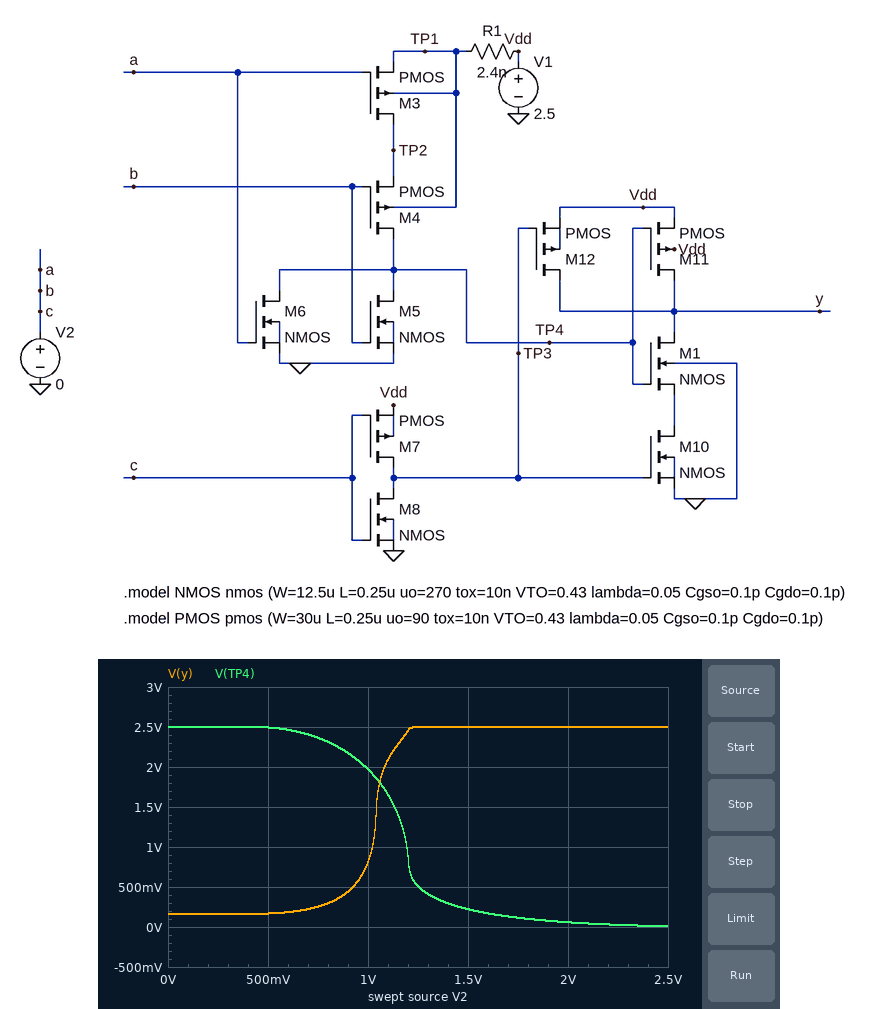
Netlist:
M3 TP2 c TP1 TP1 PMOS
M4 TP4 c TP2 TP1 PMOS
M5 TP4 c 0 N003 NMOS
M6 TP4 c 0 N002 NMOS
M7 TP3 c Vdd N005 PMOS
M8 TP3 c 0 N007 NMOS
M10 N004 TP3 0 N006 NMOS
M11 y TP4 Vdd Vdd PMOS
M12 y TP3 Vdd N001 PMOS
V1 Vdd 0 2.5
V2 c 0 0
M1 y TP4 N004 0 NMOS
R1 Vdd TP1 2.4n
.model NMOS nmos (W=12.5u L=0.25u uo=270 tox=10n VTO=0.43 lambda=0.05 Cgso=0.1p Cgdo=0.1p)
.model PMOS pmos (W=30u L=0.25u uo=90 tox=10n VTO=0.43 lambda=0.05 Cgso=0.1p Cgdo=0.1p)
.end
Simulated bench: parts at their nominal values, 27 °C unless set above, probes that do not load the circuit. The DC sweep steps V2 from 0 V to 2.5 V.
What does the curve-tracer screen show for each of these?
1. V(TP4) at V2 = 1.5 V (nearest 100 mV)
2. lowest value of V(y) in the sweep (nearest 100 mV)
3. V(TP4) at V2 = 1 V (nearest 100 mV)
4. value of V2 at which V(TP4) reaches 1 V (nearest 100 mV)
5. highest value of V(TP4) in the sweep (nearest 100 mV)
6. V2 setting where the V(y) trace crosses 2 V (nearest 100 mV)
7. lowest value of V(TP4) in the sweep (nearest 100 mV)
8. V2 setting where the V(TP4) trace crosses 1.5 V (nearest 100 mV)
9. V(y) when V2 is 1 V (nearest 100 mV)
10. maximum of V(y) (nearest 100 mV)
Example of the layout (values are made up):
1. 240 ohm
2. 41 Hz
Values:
1. 200 mV
2. 200 mV
3. 2.0 V
4. 1.2 V
5. 2.5 V
6. 1.1 V
7. 0 V
8. 1.1 V
9. 800 mV
10. 2.5 V
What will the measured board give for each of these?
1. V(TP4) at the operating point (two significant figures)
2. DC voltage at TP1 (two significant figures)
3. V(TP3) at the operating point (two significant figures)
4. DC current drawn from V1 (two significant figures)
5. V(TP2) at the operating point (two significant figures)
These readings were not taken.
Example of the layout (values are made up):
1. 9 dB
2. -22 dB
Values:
1. 2.5 V
2. 2.5 V
3. 2.5 V
4. 770 µA
5. 2.5 V
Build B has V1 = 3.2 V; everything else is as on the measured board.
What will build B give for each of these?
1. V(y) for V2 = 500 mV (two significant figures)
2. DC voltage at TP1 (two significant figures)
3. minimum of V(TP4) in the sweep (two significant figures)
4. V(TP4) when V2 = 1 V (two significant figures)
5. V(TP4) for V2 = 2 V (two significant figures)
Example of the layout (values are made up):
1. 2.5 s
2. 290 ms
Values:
1. 130 mV
2. 3.2 V
3. 67 mV
4. 2.8 V
5. 190 mV
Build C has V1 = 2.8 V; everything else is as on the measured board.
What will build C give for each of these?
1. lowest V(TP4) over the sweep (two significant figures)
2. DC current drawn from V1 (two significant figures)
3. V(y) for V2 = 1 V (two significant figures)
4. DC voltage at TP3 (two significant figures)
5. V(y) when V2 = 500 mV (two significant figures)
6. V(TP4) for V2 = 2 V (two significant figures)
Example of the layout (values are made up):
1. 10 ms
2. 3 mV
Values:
1. 28 mV
2. 780 µA
3. 510 mV
4. 2.8 V
5. 150 mV
6. 110 mV
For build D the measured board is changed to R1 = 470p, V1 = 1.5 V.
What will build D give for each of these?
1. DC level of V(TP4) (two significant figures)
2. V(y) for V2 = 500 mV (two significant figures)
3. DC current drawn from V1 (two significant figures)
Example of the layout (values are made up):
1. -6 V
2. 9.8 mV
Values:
1. 1.5 V
2. 360 mV
3. 730 µA
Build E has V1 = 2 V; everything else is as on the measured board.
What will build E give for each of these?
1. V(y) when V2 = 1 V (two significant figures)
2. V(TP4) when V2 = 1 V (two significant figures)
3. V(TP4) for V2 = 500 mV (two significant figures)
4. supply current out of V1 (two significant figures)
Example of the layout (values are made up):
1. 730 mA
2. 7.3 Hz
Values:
1. 1.9 V
2. 1.2 V
3. 2.0 V
4. 750 µA
